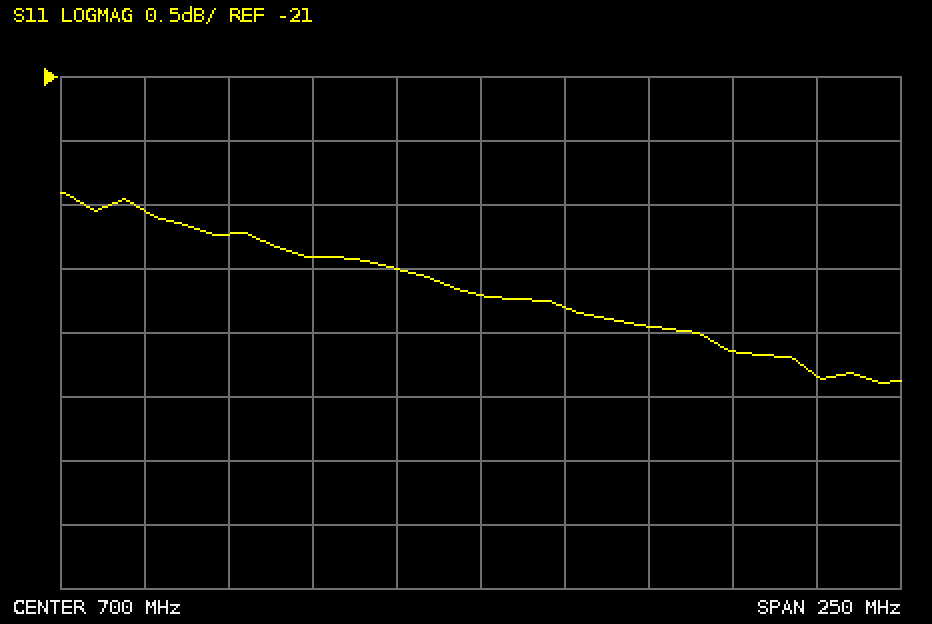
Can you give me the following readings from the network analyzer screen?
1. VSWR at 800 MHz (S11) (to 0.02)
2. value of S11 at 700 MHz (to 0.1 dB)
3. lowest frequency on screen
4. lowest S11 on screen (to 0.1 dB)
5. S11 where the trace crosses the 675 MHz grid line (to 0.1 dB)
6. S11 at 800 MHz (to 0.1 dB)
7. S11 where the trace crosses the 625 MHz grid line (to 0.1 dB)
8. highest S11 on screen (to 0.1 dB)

1.14
-22.7 dB
575 MHz
-23.4 dB
-22.5 dB
-23.3 dB
-22.2 dB
-21.9 dB
